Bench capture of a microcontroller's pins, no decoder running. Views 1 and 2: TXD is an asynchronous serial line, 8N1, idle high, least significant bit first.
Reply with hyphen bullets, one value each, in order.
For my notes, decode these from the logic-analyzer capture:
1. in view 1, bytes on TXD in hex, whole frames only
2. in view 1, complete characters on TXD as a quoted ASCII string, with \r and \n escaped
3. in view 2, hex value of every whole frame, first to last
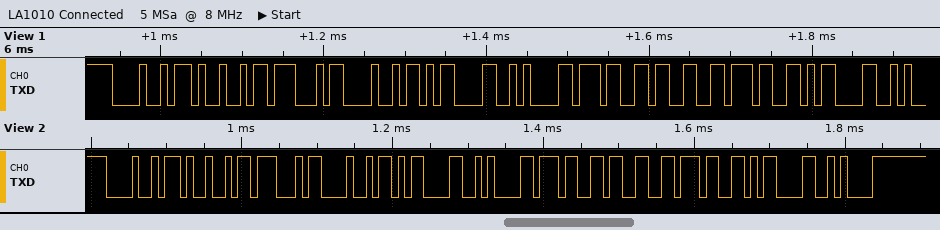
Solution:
- 48 49 47 48 0D 0A 37 33 37 0D
- "HIGH\r\n737\r"
- 48 49 47 48 0D 0A 37 33 37 0D 0A
